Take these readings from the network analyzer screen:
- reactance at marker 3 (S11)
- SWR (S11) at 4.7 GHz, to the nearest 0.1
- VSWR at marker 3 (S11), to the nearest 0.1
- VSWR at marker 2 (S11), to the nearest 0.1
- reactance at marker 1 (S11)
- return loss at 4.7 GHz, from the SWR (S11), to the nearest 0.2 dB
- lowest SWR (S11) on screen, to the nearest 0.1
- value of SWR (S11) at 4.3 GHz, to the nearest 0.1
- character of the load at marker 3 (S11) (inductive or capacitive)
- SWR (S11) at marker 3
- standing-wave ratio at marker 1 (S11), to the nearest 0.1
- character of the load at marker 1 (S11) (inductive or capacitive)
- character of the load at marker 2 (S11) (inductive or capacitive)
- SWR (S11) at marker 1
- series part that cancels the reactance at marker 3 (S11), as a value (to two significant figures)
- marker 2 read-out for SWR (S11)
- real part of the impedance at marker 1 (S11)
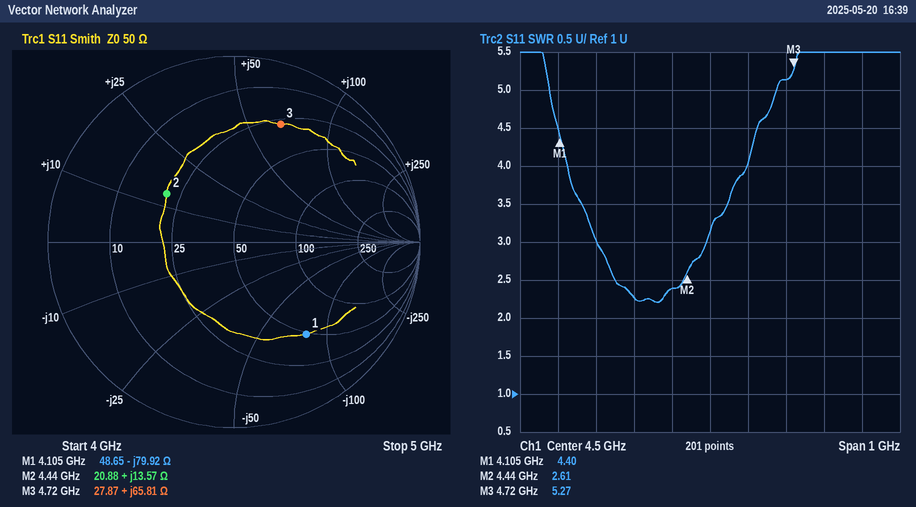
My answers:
+65.81 Ω
5.1
5.3
2.6
-79.92 Ω
3.4 dB
2.2
2.3
inductive
5.27
4.4
capacitive
inductive
4.40
510 fF
2.61
48.65 Ω
